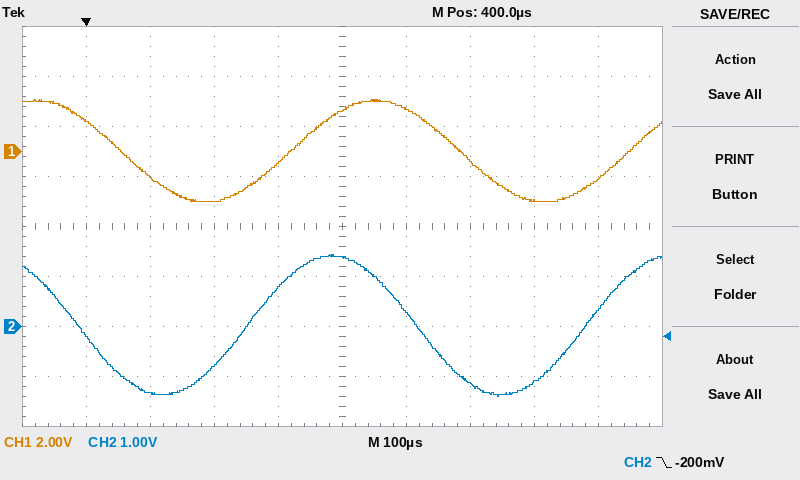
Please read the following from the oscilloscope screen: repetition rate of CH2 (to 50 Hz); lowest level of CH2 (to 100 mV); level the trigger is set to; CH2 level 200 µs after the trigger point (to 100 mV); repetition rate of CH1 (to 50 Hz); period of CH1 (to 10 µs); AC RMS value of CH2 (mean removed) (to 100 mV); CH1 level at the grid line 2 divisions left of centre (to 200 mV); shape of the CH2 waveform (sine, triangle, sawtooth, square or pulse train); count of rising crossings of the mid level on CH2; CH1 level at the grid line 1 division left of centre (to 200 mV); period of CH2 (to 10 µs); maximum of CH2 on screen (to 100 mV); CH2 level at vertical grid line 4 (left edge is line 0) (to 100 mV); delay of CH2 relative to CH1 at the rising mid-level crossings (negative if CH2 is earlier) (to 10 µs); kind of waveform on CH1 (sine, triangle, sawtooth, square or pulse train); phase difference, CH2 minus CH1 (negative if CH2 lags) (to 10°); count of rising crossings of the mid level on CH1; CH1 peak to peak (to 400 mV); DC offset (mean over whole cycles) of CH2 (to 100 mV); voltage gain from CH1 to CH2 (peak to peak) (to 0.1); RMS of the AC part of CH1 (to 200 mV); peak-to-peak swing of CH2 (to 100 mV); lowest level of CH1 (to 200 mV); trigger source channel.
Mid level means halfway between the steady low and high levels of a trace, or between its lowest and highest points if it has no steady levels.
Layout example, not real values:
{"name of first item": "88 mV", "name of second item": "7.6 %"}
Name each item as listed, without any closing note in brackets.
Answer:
{"repetition rate of CH2": "1.90 kHz", "lowest level of CH2": "-1.4 V", "level the trigger is set to": "-200 mV", "CH2 level 200 µs after the trigger point": "-800 mV", "repetition rate of CH1": "1.90 kHz", "period of CH1": "530 µs", "AC RMS value of CH2 (mean removed)": "1.0 V", "CH1 level at the grid line 2 divisions left of centre": "-2.0 V", "shape of the CH2 waveform": "sine", "count of rising crossings of the mid level on CH2": "2", "CH1 level at the grid line 1 division left of centre": "-400 mV", "period of CH2": "530 µs", "maximum of CH2 on screen": "1.4 V", "CH2 level at vertical grid line 4 (left edge is line 0)": "800 mV", "delay of CH2 relative to CH1 at the rising mid-level crossings (negative if CH2 is earlier)": "-70 µs", "kind of waveform on CH1": "sine", "phase difference, CH2 minus CH1 (negative if CH2 lags)": "+50°", "count of rising crossings of the mid level on CH1": "2", "CH1 peak to peak": "4.0 V", "DC offset (mean over whole cycles) of CH2": "0.0 V", "voltage gain from CH1 to CH2 (peak to peak)": "0.7", "RMS of the AC part of CH1": "1.4 V", "peak-to-peak swing of CH2": "2.8 V", "lowest level of CH1": "-2.0 V", "trigger source channel": "CH2"}
